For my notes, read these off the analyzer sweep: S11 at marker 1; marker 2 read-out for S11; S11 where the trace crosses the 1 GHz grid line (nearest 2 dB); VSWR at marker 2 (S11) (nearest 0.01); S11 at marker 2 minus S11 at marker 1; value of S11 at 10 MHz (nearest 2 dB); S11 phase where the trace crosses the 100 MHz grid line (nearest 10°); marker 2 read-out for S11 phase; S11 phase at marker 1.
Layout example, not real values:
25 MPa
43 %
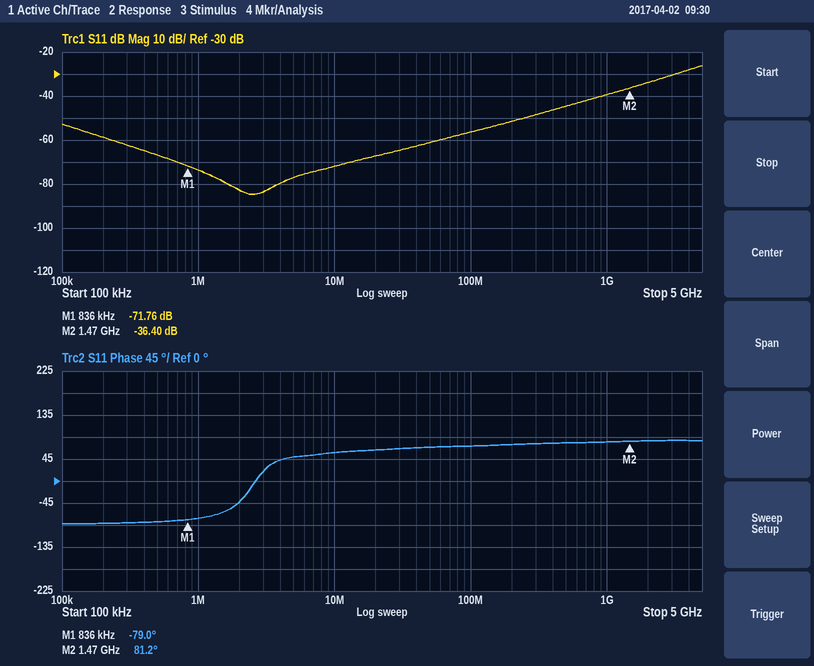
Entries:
-71.76 dB
-36.40 dB
-40 dB
1.03
35.36 dB
-72 dB
70°
81.2°
-79.0°
